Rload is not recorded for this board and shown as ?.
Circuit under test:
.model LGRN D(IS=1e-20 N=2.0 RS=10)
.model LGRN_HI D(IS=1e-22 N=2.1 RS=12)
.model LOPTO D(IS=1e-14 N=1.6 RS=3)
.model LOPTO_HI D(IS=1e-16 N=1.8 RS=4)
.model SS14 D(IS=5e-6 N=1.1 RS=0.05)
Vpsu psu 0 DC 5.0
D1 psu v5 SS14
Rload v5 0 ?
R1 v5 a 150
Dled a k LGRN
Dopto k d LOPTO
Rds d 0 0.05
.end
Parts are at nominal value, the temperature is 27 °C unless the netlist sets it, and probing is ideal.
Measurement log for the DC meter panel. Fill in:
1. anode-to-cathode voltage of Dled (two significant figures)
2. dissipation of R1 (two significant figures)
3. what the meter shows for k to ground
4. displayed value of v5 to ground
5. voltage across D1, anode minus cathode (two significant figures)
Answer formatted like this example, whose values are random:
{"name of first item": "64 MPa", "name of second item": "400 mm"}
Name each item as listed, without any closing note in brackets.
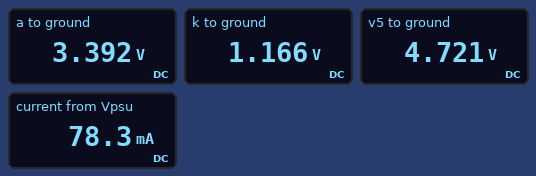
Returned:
{"anode-to-cathode voltage of Dled": "2.2 V", "dissipation of R1": "12 mW", "what the meter shows for k to ground": "1.166 V", "displayed value of v5 to ground": "4.721 V", "voltage across D1, anode minus cathode": "280 mV"}
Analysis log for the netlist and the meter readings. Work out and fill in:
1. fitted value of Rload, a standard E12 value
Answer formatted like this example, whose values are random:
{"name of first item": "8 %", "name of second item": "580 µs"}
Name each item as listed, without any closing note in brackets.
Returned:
{"fitted value of Rload, a standard E12 value": "68 Ω"}
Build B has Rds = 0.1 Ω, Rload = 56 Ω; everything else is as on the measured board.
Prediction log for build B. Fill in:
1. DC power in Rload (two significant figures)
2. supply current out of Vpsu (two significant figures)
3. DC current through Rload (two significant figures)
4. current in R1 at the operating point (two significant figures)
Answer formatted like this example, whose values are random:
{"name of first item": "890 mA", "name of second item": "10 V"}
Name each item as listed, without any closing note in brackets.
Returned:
{"DC power in Rload": "400 mW", "supply current out of Vpsu": "93 mA", "DC current through Rload": "84 mA", "current in R1 at the operating point": "8.8 mA"}
